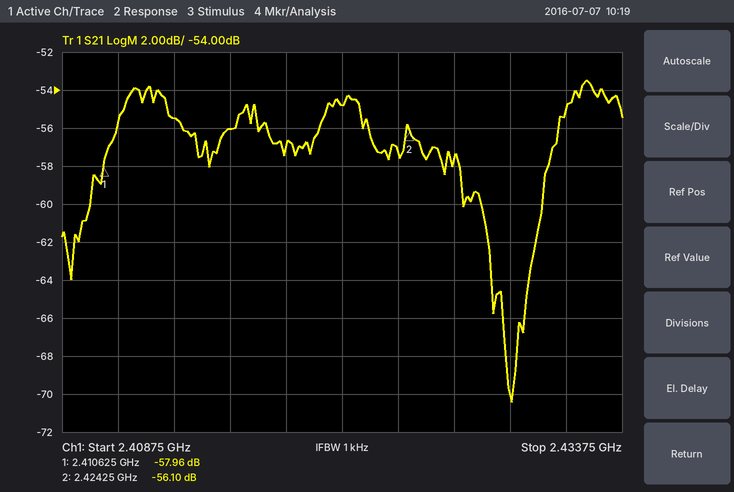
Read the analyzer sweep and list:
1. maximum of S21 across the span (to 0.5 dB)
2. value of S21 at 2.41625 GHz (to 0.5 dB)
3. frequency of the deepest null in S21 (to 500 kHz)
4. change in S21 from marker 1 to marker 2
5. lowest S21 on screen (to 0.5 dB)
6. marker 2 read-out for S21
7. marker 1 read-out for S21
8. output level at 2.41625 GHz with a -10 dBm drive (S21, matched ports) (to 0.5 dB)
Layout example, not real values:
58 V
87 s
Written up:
-53.5 dB
-56.0 dB
2.4290 GHz
1.86 dB
-70.5 dB
-56.10 dB
-57.96 dB
-66.0 dBm
